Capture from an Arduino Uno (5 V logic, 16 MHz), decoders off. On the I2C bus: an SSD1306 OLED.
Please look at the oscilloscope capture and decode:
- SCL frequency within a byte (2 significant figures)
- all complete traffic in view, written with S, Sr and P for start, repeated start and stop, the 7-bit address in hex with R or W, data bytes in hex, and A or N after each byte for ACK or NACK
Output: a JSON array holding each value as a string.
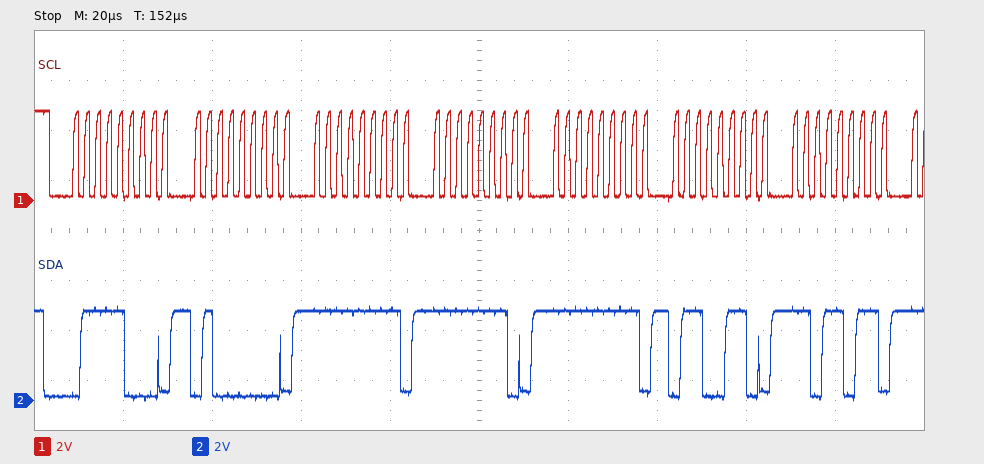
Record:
["400 kHz", "S 3CW A 40 A FF A FE A FF A 66 A DB A"]
